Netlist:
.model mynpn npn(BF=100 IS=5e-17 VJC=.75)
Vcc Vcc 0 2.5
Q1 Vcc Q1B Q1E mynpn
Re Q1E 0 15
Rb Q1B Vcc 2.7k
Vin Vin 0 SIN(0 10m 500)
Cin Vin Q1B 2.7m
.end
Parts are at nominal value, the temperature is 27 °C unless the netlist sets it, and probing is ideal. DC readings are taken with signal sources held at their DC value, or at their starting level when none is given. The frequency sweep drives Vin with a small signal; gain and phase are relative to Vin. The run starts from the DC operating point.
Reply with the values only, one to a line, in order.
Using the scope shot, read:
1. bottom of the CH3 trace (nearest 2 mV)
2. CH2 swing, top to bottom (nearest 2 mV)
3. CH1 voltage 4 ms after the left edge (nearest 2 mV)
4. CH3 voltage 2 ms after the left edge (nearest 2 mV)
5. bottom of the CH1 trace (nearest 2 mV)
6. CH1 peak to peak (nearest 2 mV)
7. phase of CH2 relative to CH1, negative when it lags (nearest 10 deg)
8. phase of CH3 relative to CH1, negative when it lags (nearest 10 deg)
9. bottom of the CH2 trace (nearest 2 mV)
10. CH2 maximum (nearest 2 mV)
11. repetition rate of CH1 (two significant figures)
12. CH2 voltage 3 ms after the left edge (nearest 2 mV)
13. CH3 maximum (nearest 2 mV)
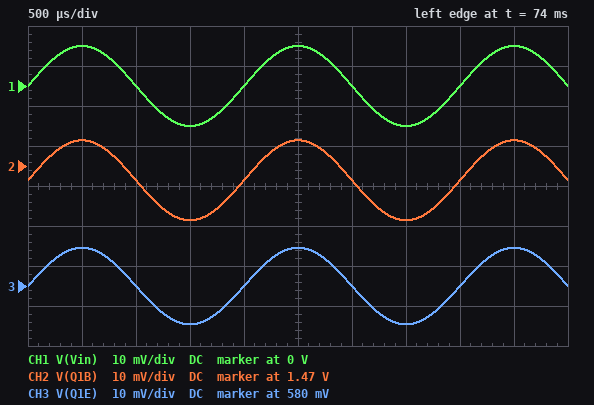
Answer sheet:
570 mV
20 mV
0 V
580 mV
-10 mV
20 mV
0 deg
0 deg
1.456 V
1.476 V
500 Hz
1.466 V
590 mV
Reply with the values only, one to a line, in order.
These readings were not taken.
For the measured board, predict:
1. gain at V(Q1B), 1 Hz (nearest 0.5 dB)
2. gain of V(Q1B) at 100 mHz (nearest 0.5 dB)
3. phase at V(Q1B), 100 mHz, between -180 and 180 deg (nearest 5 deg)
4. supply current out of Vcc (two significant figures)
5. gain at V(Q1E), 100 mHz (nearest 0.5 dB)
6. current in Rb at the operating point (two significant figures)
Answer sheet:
0 dB
-1.5 dB
30 deg
39 mA
-1.5 dB
380 µA
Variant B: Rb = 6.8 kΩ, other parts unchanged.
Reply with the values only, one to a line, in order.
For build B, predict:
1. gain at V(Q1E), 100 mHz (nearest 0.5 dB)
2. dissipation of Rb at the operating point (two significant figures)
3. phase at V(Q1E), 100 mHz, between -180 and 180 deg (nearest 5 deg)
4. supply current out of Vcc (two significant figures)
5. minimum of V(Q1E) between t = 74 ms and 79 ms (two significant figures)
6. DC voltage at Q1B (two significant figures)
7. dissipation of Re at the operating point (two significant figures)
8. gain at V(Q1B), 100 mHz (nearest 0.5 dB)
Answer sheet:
-1.5 dB
260 µW
25 deg
20 mA
290 mV
1.2 V
5.9 mW
-1.0 dB
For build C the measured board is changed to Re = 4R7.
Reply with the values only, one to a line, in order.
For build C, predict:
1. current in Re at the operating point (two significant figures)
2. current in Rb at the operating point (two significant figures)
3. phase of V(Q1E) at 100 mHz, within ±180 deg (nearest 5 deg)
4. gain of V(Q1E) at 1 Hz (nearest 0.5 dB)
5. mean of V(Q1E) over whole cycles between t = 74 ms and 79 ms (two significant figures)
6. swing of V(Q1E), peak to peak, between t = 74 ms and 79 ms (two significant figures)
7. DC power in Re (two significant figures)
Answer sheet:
51 mA
510 µA
55 deg
-1.0 dB
240 mV
18 mV
12 mW
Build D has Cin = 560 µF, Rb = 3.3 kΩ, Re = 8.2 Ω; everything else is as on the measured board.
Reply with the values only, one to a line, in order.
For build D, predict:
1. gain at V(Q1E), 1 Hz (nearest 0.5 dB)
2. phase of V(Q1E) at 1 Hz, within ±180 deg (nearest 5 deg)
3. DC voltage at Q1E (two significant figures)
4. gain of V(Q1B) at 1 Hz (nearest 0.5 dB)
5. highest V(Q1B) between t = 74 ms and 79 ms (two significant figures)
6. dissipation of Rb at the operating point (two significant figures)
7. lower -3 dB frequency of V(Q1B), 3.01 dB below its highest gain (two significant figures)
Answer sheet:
-1.5 dB
20 deg
320 mV
-0.5 dB
1.2 V
500 µW
400 mHz
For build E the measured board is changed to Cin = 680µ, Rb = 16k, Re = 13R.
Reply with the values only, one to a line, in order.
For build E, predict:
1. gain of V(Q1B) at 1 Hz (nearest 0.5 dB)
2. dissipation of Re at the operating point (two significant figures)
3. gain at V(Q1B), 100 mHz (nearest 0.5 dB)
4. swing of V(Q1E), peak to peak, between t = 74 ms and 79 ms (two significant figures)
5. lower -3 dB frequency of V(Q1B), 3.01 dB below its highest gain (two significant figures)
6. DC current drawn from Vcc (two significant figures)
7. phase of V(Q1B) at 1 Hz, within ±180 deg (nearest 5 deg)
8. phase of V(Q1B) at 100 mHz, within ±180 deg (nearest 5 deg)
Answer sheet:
0 dB
1.2 mW
-5.5 dB
17 mV
160 mHz
9.6 mA
10 deg
60 deg
